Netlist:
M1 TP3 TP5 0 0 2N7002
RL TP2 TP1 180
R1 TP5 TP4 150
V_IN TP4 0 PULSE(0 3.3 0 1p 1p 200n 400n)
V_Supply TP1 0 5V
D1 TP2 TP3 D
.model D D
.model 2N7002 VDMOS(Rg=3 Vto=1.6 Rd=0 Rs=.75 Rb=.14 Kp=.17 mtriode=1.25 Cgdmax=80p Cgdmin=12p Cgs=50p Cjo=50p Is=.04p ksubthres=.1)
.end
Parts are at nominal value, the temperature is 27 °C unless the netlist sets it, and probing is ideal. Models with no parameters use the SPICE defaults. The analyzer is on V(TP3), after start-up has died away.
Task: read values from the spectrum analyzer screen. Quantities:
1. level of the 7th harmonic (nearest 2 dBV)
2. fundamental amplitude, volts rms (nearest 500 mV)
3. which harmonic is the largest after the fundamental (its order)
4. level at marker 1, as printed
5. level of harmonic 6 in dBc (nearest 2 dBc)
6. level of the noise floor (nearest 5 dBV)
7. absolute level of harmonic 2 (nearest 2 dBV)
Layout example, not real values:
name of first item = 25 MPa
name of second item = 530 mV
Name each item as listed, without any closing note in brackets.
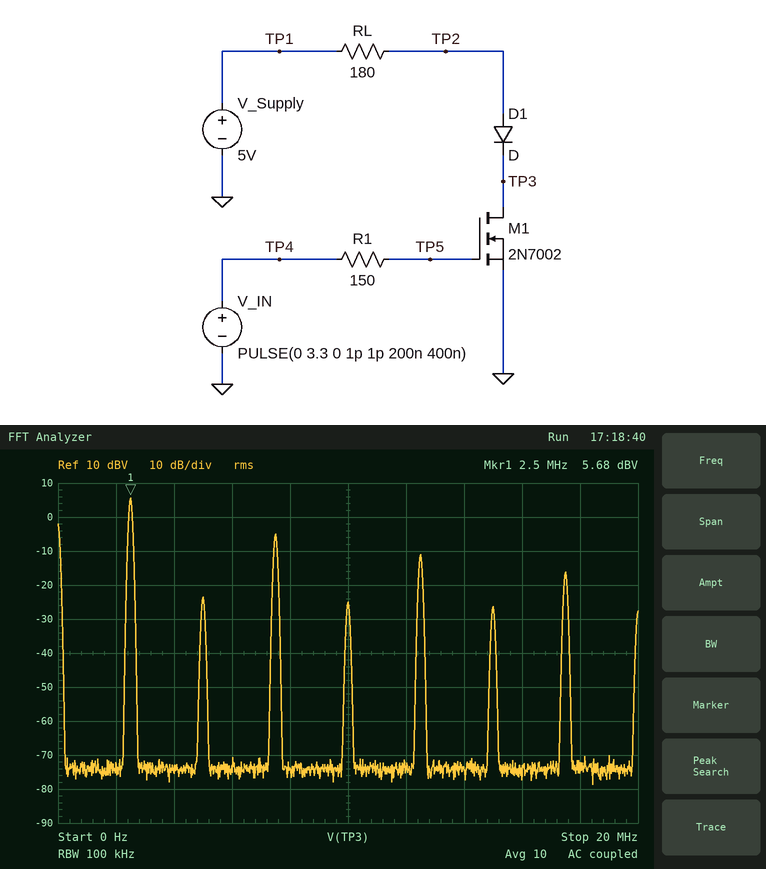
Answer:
level of the 7th harmonic = -16 dBV
fundamental amplitude, volts rms = 2.0 V
which harmonic is the largest after the fundamental = 3
level at marker 1, as printed = 5.68 dBV
level of harmonic 6 in dBc = -32 dBc
level of the noise floor = -75 dBV
absolute level of harmonic 2 = -24 dBV
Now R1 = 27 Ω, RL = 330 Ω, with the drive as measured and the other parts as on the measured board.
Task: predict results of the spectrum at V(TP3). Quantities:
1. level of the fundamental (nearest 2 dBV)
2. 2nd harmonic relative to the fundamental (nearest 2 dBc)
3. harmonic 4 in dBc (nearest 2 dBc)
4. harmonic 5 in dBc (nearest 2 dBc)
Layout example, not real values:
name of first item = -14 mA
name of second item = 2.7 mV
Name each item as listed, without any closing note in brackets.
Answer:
level of the fundamental = 6 dBV
2nd harmonic relative to the fundamental = -14 dBc
harmonic 4 in dBc = -16 dBc
harmonic 5 in dBc = -18 dBc
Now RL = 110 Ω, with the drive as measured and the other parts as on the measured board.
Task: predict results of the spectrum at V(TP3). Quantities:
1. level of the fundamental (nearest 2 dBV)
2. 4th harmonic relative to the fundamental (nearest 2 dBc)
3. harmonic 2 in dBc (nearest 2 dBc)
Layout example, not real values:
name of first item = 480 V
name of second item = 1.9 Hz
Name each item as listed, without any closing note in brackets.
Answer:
level of the fundamental = 6 dBV
4th harmonic relative to the fundamental = -38 dBc
harmonic 2 in dBc = -34 dBc
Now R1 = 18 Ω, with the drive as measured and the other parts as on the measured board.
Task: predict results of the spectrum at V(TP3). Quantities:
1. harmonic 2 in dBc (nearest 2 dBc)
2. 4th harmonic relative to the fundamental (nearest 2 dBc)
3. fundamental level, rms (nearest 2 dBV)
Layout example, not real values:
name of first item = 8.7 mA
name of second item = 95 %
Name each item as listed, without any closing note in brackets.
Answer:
harmonic 2 in dBc = -20 dBc
4th harmonic relative to the fundamental = -20 dBc
fundamental level, rms = 6 dBV
